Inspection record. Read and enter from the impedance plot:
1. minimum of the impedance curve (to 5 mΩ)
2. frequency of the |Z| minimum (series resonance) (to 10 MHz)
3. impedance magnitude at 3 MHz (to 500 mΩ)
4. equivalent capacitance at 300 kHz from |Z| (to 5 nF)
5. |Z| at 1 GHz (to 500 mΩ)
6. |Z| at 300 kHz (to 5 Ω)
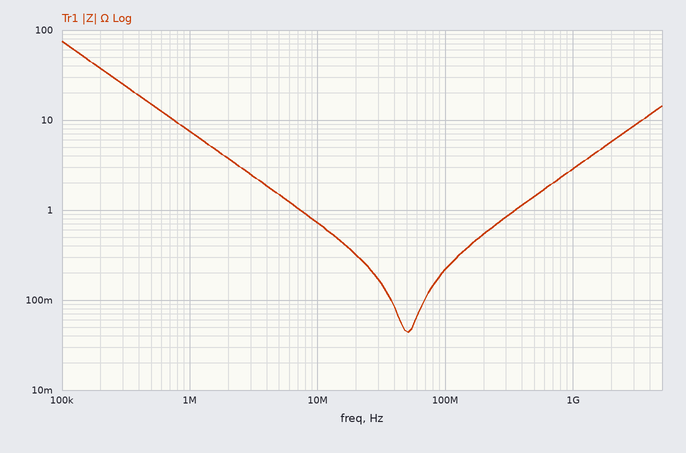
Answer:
45 mΩ
50 MHz
2.5 Ω
20 nF
3.0 Ω
25 Ω
